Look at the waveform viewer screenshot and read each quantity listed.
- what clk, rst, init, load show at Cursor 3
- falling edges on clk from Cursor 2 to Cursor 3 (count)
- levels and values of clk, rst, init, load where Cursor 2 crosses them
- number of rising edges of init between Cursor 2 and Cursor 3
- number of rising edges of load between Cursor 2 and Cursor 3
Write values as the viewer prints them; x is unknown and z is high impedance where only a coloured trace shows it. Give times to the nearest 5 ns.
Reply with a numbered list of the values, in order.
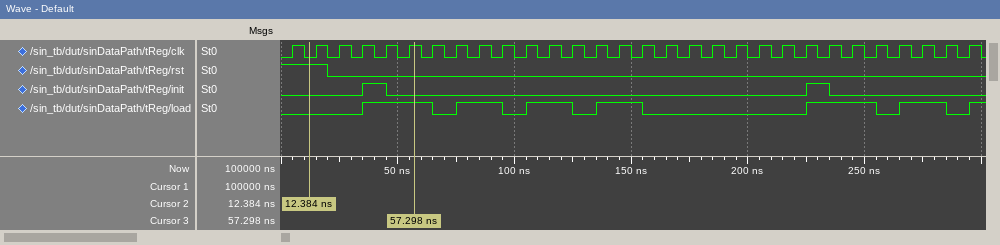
1. clk=1, rst=0, init=0, load=1
2. 4
3. clk=0, rst=1, init=0, load=0
4. 1
5. 1
